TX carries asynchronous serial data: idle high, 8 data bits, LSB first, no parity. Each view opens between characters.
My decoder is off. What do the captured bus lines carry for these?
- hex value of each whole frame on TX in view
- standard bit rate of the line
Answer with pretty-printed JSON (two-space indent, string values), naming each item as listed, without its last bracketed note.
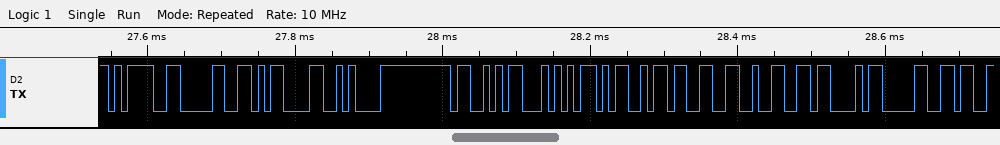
{
  "hex value of each whole frame on TX in view": "3D, 30, 0D, 0A, 53, 54, 4D, 33, 32, 43, 30",
  "standard bit rate of the line": "115200 baud"
}
